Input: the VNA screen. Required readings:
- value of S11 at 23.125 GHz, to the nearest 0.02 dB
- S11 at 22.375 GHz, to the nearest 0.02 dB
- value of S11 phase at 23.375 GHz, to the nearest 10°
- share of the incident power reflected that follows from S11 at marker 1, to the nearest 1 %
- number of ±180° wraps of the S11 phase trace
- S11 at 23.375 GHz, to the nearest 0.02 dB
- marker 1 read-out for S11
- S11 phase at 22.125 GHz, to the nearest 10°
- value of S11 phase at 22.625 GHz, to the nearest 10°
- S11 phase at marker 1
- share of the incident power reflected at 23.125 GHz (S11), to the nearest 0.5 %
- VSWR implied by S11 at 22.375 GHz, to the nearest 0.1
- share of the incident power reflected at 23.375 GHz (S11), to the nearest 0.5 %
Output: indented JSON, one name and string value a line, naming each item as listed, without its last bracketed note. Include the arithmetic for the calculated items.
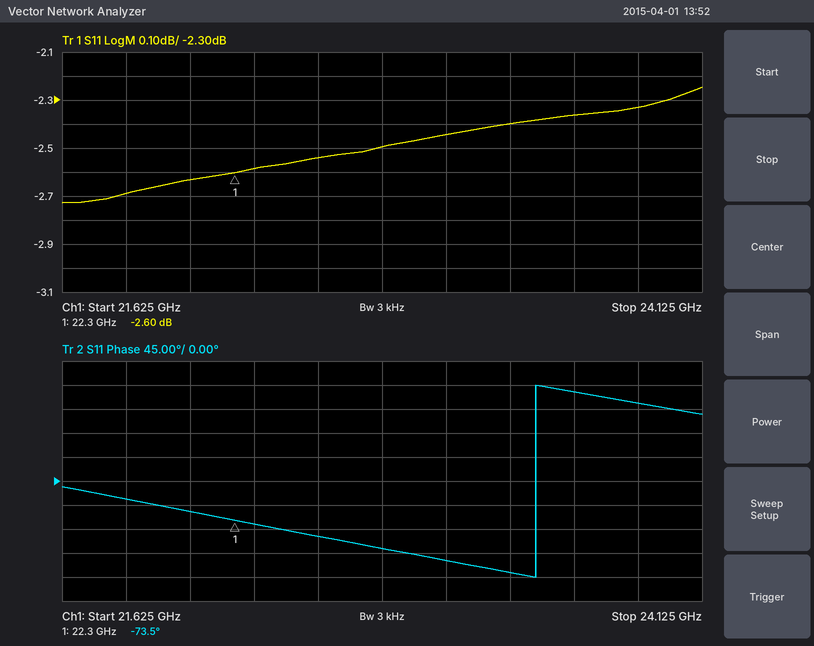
{
  "value of S11 at 23.125 GHz, to the nearest 0.02 dB": "-2.44 dB",
  "S11 at 22.375 GHz, to the nearest 0.02 dB": "-2.58 dB",
  "value of S11 phase at 23.375 GHz, to the nearest 10°": "-170°",
  "share of the incident power reflected that follows from S11 at marker 1, to the nearest 1 %": "10^(-2.6/10) ≈ 55 %",
  "number of ±180° wraps of the S11 phase trace": "1",
  "S11 at 23.375 GHz, to the nearest 0.02 dB": "-2.40 dB",
  "marker 1 read-out for S11": "-2.60 dB",
  "S11 phase at 22.125 GHz, to the nearest 10°": "-60°",
  "value of S11 phase at 22.625 GHz, to the nearest 10°": "-100°",
  "S11 phase at marker 1": "-73.5°",
  "share of the incident power reflected at 23.125 GHz (S11), to the nearest 0.5 %": "10^(-2.44/10) ≈ 57.0 %",
  "VSWR implied by S11 at 22.375 GHz, to the nearest 0.1": "|Γ| = 10^(-2.58/20) = 0.7430; VSWR = (1 + 0.7430)/(1 − 0.7430) ≈ 6.8",
  "share of the incident power reflected at 23.375 GHz (S11), to the nearest 0.5 %": "10^(-2.4/10) ≈ 57.5 %"
}
